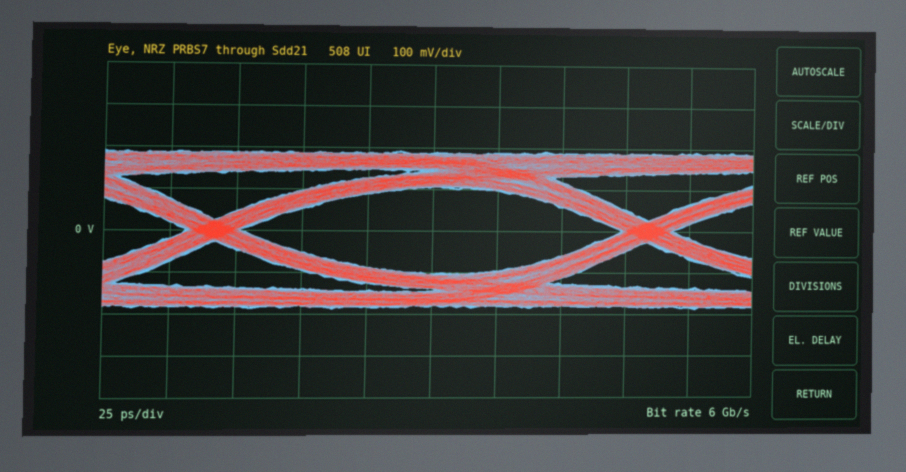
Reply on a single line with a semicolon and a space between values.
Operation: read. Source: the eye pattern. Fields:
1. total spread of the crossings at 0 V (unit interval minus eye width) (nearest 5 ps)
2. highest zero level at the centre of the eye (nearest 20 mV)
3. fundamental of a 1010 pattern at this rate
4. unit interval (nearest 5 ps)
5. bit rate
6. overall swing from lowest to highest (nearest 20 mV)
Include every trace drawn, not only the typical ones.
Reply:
20 ps; -100 mV; 3 GHz; 165 ps; 6 Gb/s; 380 mV
